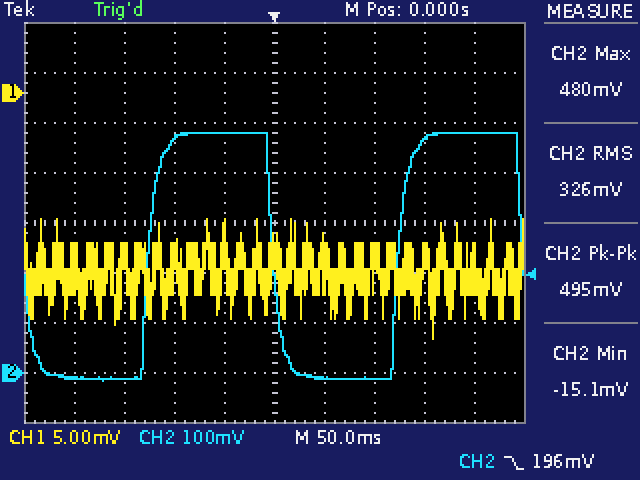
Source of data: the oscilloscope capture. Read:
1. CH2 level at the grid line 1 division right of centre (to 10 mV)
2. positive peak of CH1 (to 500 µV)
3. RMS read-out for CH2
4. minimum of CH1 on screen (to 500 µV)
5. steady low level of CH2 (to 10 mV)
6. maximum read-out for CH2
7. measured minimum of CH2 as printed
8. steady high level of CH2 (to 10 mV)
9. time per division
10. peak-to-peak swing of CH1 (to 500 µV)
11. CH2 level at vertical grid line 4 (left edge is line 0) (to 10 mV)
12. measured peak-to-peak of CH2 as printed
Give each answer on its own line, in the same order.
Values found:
-10 mV
-12.5 mV
326 mV
-24.5 mV
-10 mV
480 mV
-15.1 mV
480 mV
50 ms
12.0 mV
480 mV
495 mV
